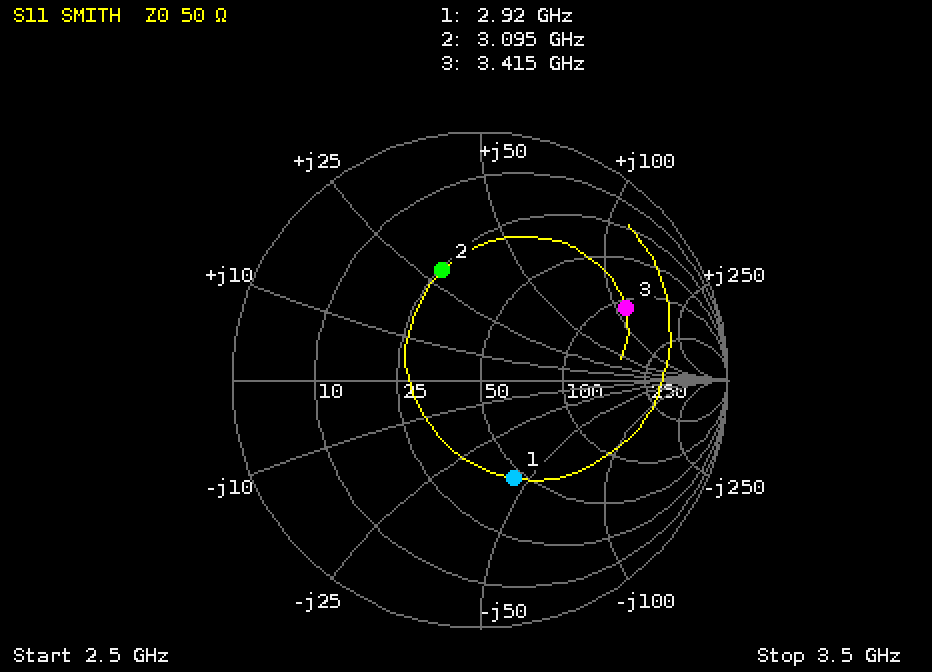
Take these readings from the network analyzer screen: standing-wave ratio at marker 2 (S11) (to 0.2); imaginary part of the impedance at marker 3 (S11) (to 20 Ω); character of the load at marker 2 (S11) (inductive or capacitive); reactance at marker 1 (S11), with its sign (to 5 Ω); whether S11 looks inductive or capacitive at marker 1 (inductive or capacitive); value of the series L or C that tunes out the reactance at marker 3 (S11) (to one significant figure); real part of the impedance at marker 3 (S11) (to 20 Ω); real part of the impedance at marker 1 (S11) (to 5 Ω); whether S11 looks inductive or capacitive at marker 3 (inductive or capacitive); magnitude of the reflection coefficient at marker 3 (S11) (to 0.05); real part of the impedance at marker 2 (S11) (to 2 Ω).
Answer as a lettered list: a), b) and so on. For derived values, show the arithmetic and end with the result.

a) 2.8
b) +120 Ω
c) inductive
d) -45 Ω
e) capacitive
f) C = 1/(2π × 3.415 GHz × 120 Ω) ≈ 388 fF, so 400 fF to one significant figure
g) 120 Ω
h) 45 Ω
i) inductive
j) 0.65
k) 26 Ω
